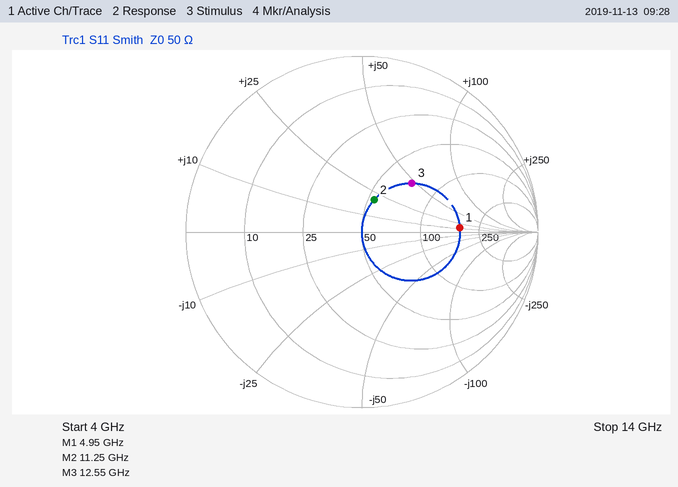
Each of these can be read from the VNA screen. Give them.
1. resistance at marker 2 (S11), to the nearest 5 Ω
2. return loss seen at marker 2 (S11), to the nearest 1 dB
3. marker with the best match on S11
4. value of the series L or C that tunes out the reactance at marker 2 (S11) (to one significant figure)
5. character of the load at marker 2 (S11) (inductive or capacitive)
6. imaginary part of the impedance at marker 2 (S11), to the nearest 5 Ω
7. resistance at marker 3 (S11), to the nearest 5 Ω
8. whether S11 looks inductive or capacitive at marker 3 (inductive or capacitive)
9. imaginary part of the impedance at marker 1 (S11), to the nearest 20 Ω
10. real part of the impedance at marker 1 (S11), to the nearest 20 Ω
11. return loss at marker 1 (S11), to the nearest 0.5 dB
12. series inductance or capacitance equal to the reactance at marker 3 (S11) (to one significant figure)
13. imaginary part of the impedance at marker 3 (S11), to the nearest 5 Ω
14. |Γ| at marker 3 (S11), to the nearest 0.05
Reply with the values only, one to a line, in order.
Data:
55 Ω
14 dB
marker 2
700 fF
inductive
+20 Ω
70 Ω
inductive
+20 Ω
180 Ω
5.0 dB
600 pH
+45 Ω
0.40
